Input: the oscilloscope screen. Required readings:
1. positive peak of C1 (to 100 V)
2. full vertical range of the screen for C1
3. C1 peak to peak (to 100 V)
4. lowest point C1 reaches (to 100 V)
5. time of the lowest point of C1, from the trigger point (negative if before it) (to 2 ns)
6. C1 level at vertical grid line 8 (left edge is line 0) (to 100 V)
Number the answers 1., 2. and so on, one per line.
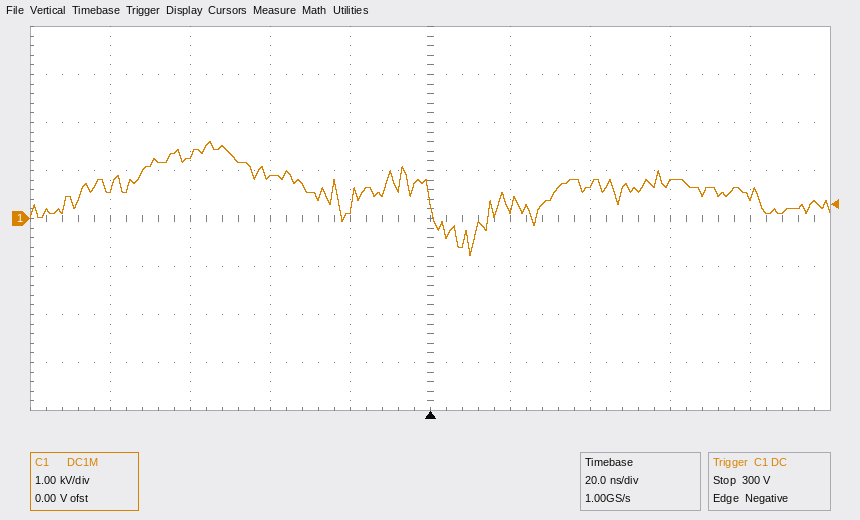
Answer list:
1. 1.6 kV
2. 8 kV
3. 2.4 kV
4. -800 V
5. +10 ns
6. 700 V
